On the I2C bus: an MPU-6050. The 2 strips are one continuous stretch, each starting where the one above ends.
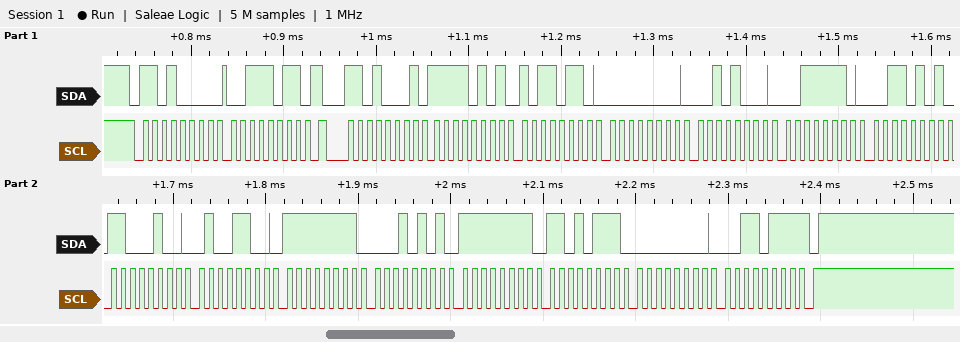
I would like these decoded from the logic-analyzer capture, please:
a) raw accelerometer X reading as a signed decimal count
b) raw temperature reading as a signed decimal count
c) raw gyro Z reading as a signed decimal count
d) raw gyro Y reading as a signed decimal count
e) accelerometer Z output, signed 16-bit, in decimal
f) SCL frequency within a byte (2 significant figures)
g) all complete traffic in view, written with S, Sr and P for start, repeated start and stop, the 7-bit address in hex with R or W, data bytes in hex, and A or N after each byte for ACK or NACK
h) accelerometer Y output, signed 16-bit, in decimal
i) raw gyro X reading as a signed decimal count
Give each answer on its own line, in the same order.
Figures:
-2634
-15284
55
-41
15925
100 kHz
S 68W A 3B A Sr 68R A F5 A B6 A 00 A 28 A 3E A 35 A C4 A 4C A FF A 15 A FF A D7 A 00 A 37 N P
40
-235
